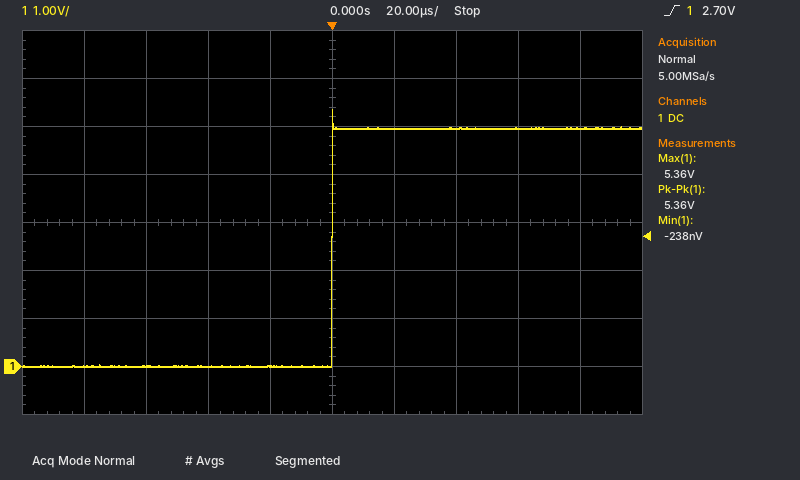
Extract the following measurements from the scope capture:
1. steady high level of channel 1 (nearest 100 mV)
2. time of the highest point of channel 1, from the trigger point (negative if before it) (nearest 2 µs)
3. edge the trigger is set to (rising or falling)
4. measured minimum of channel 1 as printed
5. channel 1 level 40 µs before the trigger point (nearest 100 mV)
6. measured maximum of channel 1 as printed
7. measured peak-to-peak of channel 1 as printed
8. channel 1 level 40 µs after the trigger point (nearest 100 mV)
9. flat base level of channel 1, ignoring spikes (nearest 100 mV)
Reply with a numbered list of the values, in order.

1. 5.0 V
2. 0 µs
3. rising
4. -238 nV
5. 0.0 V
6. 5.36 V
7. 5.36 V
8. 5.0 V
9. 0.0 V
